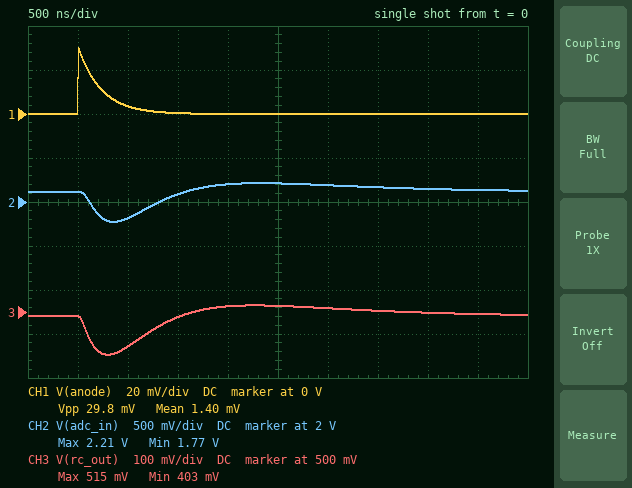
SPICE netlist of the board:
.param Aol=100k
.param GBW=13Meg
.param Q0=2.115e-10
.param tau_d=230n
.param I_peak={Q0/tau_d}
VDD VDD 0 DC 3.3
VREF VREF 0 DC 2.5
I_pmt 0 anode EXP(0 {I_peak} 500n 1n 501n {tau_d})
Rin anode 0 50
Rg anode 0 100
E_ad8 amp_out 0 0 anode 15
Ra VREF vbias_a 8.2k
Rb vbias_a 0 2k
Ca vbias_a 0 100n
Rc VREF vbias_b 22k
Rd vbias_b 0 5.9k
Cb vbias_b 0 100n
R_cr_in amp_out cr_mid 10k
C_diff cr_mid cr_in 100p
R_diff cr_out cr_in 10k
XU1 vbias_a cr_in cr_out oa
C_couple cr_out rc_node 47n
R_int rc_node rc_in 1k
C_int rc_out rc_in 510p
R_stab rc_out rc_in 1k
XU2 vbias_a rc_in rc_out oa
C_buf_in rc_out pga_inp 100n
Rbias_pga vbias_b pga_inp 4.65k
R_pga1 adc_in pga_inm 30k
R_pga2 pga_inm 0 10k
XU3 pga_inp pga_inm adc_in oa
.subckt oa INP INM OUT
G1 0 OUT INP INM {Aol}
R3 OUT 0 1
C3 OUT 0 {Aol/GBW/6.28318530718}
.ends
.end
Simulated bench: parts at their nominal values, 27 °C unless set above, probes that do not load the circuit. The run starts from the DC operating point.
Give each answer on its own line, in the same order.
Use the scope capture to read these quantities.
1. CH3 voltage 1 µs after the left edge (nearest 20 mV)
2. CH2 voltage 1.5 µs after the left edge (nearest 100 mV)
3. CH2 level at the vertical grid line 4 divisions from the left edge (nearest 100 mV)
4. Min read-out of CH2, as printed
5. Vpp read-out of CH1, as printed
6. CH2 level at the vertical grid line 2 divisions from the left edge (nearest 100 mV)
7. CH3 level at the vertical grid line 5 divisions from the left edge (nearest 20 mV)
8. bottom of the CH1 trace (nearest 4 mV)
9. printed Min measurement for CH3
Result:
420 mV
2.1 V
2.2 V
1.77 V
29.8 mV
1.8 V
520 mV
0 V
403 mV
